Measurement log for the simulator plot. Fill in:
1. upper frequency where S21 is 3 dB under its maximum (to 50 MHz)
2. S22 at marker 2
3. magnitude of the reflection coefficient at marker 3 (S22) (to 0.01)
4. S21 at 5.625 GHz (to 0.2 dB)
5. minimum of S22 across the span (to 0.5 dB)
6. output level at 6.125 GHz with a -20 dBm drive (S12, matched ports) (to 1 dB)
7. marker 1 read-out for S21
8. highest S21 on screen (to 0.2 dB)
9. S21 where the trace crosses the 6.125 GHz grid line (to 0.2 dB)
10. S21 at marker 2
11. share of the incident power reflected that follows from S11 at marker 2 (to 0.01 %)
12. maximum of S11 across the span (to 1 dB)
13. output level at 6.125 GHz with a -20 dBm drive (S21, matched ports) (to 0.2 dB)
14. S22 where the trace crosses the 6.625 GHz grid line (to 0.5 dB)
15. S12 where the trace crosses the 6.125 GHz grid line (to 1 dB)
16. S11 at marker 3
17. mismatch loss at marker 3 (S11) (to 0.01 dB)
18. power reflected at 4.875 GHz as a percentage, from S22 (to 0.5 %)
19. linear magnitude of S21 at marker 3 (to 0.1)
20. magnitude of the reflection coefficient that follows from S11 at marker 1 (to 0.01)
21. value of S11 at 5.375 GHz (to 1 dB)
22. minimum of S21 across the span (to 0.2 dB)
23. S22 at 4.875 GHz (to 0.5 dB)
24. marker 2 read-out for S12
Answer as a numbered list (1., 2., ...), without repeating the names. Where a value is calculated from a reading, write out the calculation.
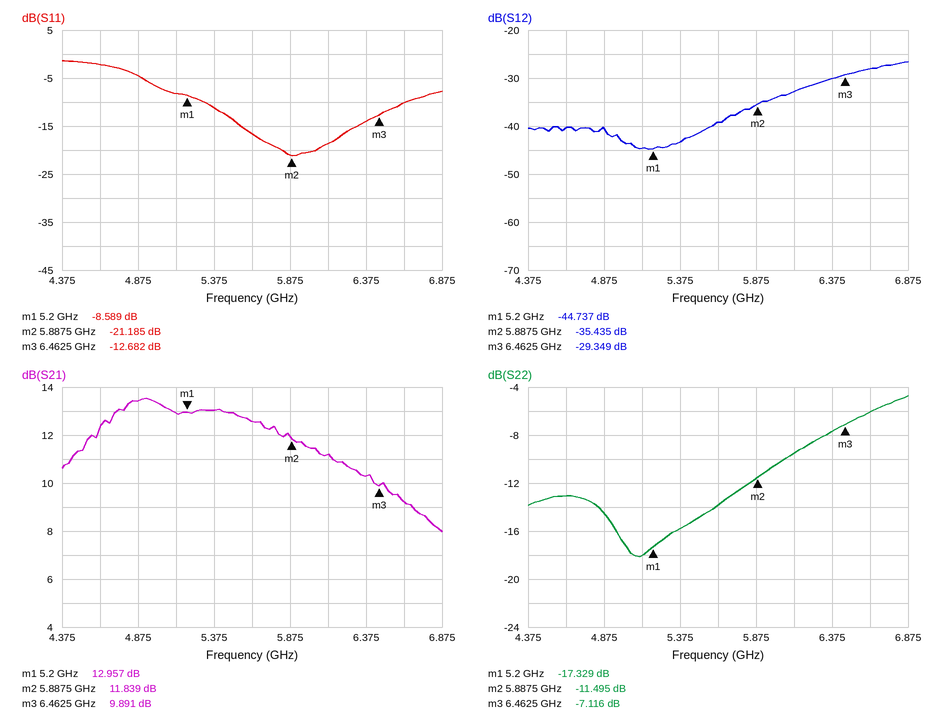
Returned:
1. 6.30 GHz
2. -11.495 dB
3. 10^(-7.116/20) ≈ 0.44
4. 12.6 dB
5. -18.0 dB
6. -20 dBm + (-33 dB) = -53 dBm
7. 12.957 dB
8. 13.6 dB
9. 11.2 dB
10. 11.839 dB
11. 10^(-21.185/10) ≈ 0.76 %
12. -1 dB
13. -20 dBm + (11.2 dB) = -8.8 dBm
14. -6.0 dB
15. -33 dB
16. -12.682 dB
17. −10 log10(1 − 10^(-12.682/10)) ≈ 0.24 dB
18. 10^(-14.5/10) ≈ 3.5 %
19. 10^(9.891/20) ≈ 3.1
20. 10^(-8.589/20) ≈ 0.37
21. -11 dB
22. 8.0 dB
23. -14.5 dB
24. -35.435 dB
